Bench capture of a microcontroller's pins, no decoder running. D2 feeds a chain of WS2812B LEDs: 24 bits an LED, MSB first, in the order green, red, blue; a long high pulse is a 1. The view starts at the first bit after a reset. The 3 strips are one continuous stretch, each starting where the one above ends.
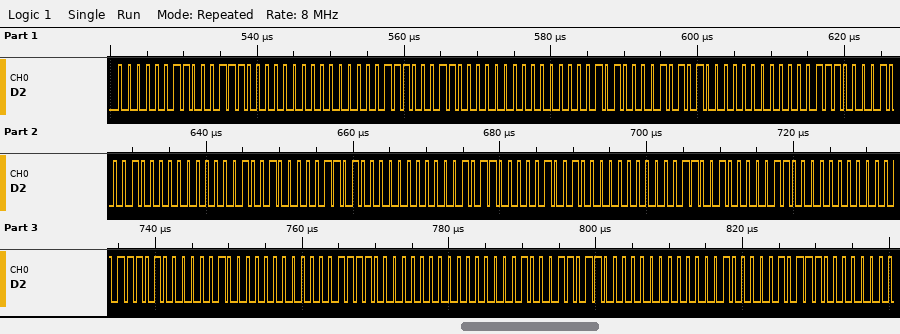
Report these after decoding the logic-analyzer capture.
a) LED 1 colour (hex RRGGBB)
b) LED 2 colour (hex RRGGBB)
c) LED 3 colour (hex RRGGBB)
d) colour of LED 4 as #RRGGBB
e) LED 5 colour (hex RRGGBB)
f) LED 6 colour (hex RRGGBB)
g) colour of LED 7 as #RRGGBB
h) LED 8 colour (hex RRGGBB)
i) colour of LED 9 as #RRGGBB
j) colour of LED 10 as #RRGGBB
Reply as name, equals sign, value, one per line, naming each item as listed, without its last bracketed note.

LED 1 colour = #1C0300
LED 2 colour = #180700
LED 3 colour = #150A00
colour of LED 4 as #RRGGBB = #110E00
LED 5 colour = #0D1200
LED 6 colour = #091600
colour of LED 7 as #RRGGBB = #061900
LED 8 colour = #021D00
colour of LED 9 as #RRGGBB = #001E01
colour of LED 10 as #RRGGBB = #001B04
